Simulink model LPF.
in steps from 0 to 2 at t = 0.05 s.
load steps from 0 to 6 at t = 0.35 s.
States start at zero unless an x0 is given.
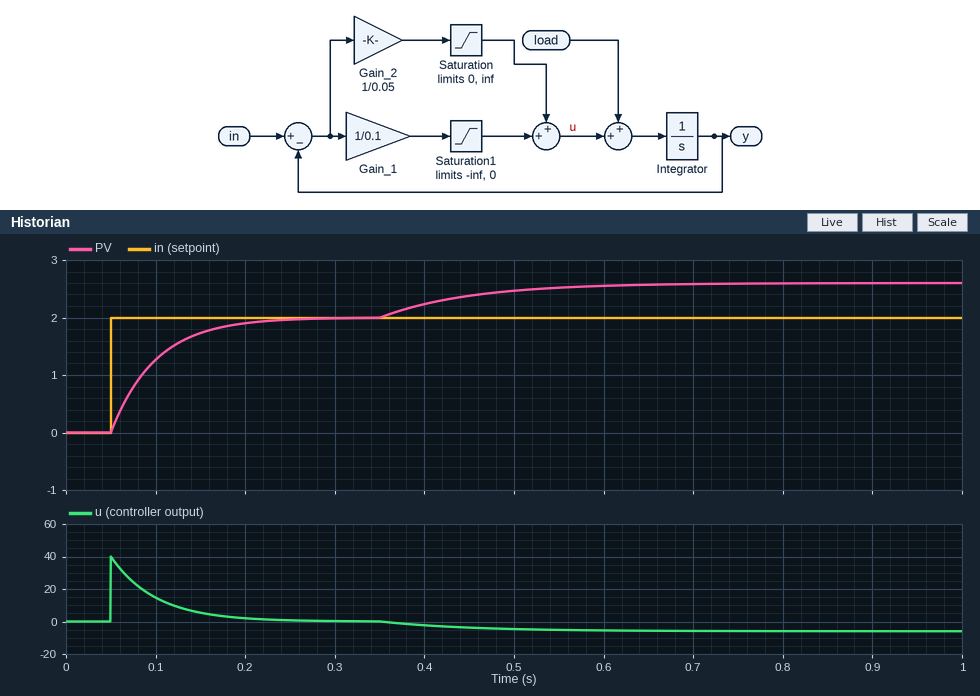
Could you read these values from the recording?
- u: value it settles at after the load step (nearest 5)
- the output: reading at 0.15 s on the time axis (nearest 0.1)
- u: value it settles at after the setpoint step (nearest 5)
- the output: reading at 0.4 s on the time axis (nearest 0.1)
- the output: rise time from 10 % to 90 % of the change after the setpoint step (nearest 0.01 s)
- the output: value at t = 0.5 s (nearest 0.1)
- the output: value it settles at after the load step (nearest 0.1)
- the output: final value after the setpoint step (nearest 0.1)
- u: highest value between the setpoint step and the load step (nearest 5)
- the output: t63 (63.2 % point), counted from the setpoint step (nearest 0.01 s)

-5
1.7
0
2.2
0.11 s
2.5
2.6
2.0
40
0.05 s
